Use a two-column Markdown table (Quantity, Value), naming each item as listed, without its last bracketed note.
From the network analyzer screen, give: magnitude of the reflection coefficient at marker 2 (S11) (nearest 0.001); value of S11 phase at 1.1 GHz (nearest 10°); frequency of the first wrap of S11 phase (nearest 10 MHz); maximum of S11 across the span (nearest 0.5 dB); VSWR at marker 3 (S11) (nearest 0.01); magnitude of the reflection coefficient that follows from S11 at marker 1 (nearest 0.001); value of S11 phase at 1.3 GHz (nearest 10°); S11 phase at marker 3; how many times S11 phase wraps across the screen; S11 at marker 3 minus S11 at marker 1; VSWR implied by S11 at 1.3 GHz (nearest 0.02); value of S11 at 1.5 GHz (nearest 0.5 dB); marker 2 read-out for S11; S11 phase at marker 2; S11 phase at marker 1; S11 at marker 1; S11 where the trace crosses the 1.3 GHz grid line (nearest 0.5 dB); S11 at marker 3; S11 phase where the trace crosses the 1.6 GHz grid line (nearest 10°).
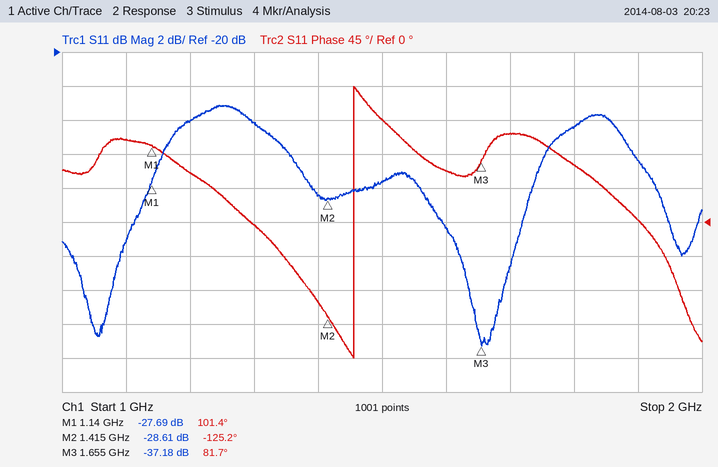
| Quantity | Value |
|---|---|
| magnitude of the reflection coefficient at marker 2 (S11) | 0.037 |
| value of S11 phase at 1.1 GHz | 110° |
| frequency of the first wrap of S11 phase | 1.46 GHz |
| maximum of S11 across the span | -23.0 dB |
| VSWR at marker 3 (S11) | 1.03 |
| magnitude of the reflection coefficient that follows from S11 at marker 1 | 0.041 |
| value of S11 phase at 1.3 GHz | 0° |
| S11 phase at marker 3 | 81.7° |
| how many times S11 phase wraps across the screen | 1 |
| S11 at marker 3 minus S11 at marker 1 | -9.49 dB |
| VSWR implied by S11 at 1.3 GHz | 1.14 |
| value of S11 at 1.5 GHz | -27.5 dB |
| marker 2 read-out for S11 | -28.61 dB |
| S11 phase at marker 2 | -125.2° |
| S11 phase at marker 1 | 101.4° |
| S11 at marker 1 | -27.69 dB |
| S11 where the trace crosses the 1.3 GHz grid line | -24.0 dB |
| S11 at marker 3 | -37.18 dB |
| S11 phase where the trace crosses the 1.6 GHz grid line | 70° |
